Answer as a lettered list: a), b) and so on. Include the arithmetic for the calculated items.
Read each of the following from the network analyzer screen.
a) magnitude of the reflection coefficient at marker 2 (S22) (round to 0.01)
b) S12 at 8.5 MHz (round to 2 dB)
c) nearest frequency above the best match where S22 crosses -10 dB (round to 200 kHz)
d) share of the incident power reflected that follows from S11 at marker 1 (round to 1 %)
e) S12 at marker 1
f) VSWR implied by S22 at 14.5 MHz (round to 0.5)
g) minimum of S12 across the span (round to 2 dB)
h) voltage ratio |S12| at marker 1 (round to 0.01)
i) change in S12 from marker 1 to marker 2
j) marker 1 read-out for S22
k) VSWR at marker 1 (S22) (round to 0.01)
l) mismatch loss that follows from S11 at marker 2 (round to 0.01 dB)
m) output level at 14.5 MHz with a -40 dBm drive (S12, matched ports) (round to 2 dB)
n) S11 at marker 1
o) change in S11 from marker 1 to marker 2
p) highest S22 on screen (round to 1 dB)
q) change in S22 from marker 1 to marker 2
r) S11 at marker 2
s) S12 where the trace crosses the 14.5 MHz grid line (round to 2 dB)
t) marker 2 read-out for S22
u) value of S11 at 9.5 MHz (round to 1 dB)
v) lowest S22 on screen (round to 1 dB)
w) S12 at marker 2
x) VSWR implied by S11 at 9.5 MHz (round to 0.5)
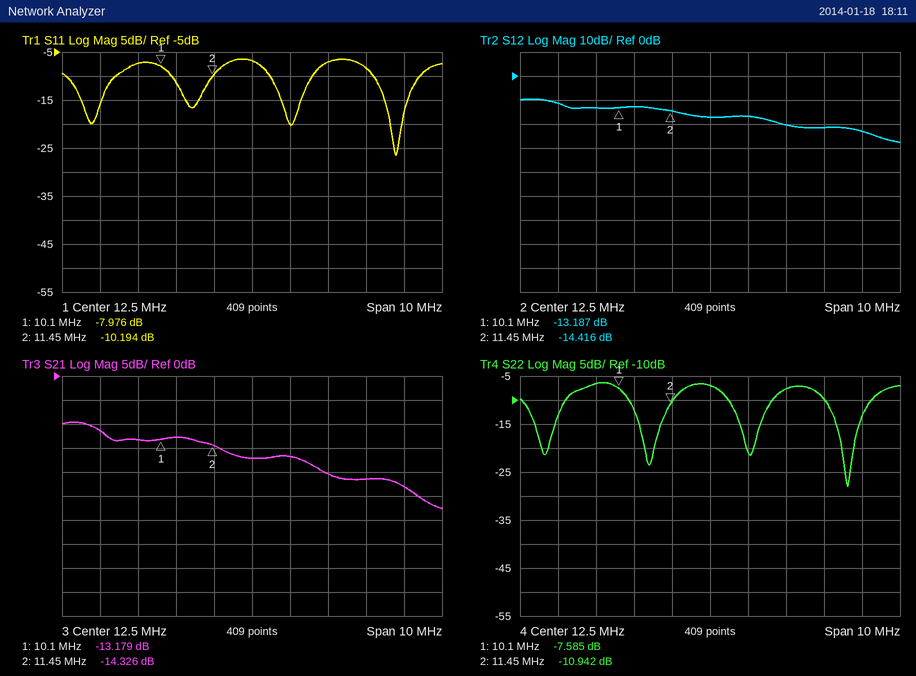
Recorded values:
a) 10^(-10.942/20) ≈ 0.28
b) -12 dB
c) 16.8 MHz
d) 10^(-7.976/10) ≈ 16 %
e) -13.187 dB
f) |Γ| = 10^(-8/20) = 0.3981; VSWR = (1 + 0.3981)/(1 − 0.3981) ≈ 2.32, so 2.5 to the nearest 0.5
g) -28 dB
h) 10^(-13.187/20) ≈ 0.22
i) -14.416 − (-13.187) = -1.229 dB
j) -7.585 dB
k) (1 + 0.4176)/(1 − 0.4176) ≈ 2.43
l) −10 log10(1 − 10^(-10.194/10)) ≈ 0.44 dB
m) -40 dBm + (-20 dB) = -60 dBm
n) -7.976 dB
o) -10.194 − (-7.976) = -2.218 dB
p) -6 dB
q) -10.942 − (-7.585) = -3.357 dB
r) -10.194 dB
s) -20 dB
t) -10.942 dB
u) -7 dB
v) -28 dB
w) -14.416 dB
x) |Γ| = 10^(-7/20) = 0.4467; VSWR = (1 + 0.4467)/(1 − 0.4467) ≈ 2.61, so 2.5 to the nearest 0.5
